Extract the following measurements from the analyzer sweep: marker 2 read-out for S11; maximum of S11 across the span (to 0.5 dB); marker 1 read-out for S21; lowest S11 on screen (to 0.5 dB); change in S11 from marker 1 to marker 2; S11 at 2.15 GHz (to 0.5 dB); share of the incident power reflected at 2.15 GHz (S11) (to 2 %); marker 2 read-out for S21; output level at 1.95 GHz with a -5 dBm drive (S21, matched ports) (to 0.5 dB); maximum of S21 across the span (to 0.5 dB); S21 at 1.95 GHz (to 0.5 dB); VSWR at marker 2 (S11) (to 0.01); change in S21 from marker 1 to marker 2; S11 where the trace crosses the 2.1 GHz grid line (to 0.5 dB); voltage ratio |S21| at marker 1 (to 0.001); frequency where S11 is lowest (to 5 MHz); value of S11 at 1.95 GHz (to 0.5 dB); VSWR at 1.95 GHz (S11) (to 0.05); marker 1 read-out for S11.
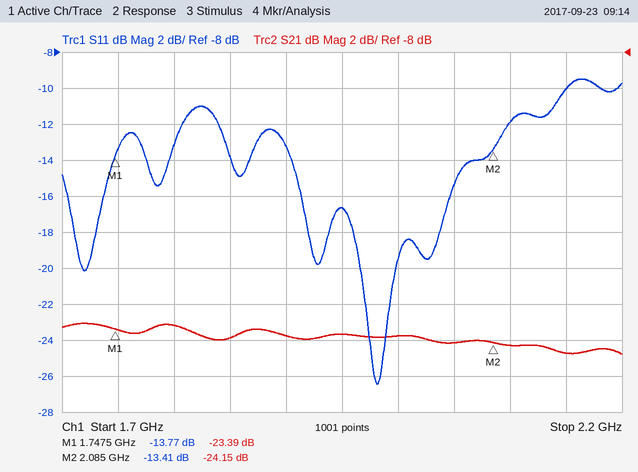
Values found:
-13.41 dB
-9.5 dB
-23.39 dB
-26.5 dB
0.36 dB
-10.0 dB
10 %
-24.15 dB
-28.5 dBm
-23.0 dB
-23.5 dB
1.54
-0.76 dB
-12.0 dB
0.068
1.980 GHz
-16.5 dB
1.35
-13.77 dB
